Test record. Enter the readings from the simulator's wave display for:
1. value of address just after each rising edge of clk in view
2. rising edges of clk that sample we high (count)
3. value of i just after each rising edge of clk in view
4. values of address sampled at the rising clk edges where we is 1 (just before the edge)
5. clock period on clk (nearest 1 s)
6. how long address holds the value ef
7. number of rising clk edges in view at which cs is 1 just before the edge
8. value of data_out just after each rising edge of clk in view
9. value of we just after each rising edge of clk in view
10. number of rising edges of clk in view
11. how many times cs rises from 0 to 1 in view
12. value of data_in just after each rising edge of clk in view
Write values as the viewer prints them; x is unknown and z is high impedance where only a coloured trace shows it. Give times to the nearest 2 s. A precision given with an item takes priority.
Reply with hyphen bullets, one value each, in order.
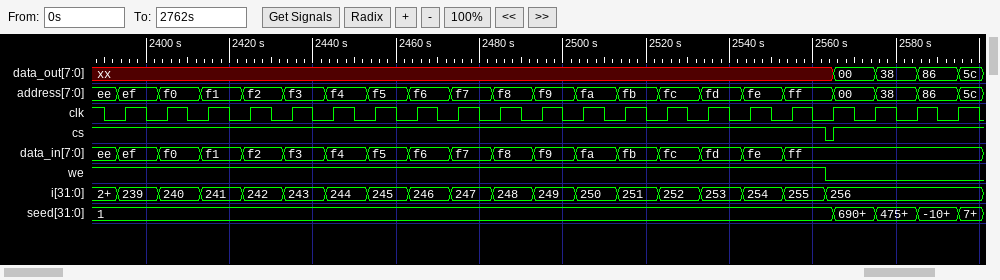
- ef, f0, f1, f2, f3, f4, f5, f6, f7, f8, f9, fa, fb, fc, fd, fe, ff, 00, 38, 86, 5c
- 17
- 239, 240, 241, 242, 243, 244, 245, 246, 247, 248, 249, 250, 251, 252, 253, 254, 255, 256, 256, 256, 256
- ef, f0, f1, f2, f3, f4, f5, f6, f7, f8, f9, fa, fb, fc, fd, fe, ff
- 10 s
- 10 s
- 20
- xx, xx, xx, xx, xx, xx, xx, xx, xx, xx, xx, xx, xx, xx, xx, xx, xx, 00, 38, 86, 5c
- 1 1 1 1 1 1 1 1 1 1 1 1 1 1 1 1 1 0 0 0 0
- 21
- 1
- ef, f0, f1, f2, f3, f4, f5, f6, f7, f8, f9, fa, fb, fc, fd, fe, ff, ff, ff, ff, ff
